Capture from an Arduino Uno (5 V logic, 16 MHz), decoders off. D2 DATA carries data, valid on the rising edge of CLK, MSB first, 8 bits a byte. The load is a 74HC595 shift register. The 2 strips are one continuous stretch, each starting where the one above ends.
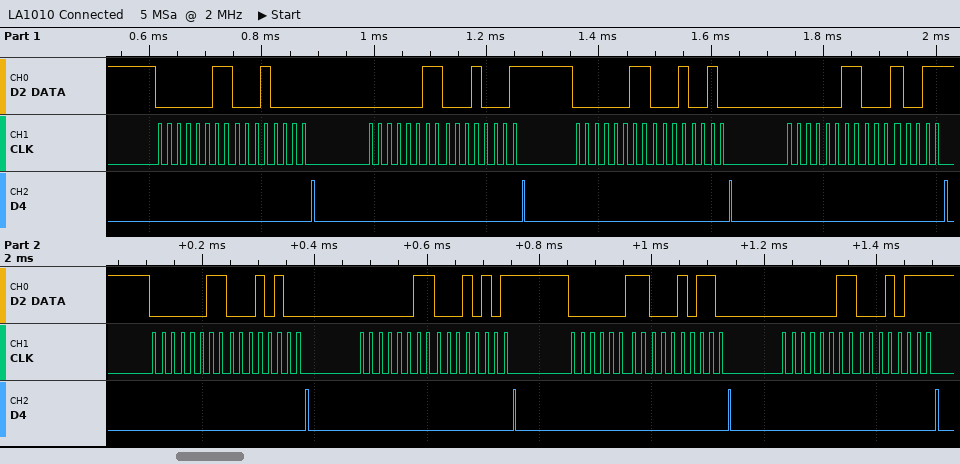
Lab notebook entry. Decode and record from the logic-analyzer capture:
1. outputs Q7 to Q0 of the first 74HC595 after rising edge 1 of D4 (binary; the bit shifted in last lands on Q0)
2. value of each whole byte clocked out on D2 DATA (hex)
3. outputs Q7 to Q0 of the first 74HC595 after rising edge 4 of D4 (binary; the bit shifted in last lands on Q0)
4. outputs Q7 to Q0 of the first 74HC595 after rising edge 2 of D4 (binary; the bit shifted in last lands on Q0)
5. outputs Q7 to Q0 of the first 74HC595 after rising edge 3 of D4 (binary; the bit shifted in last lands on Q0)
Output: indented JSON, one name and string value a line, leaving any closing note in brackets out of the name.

{
  "outputs Q7 to Q0 of the first 74HC595 after rising edge 1 of D4": "00010000",
  "value of each whole byte clocked out on D2 DATA": "0x03 0x10 0x03 0x11 0x03 0x12 0x03 0x13 0x03 0x14 0x03 0x15 0x03 0x16 0x03 0x17",
  "outputs Q7 to Q0 of the first 74HC595 after rising edge 4 of D4": "00010011",
  "outputs Q7 to Q0 of the first 74HC595 after rising edge 2 of D4": "00010001",
  "outputs Q7 to Q0 of the first 74HC595 after rising edge 3 of D4": "00010010"
}
